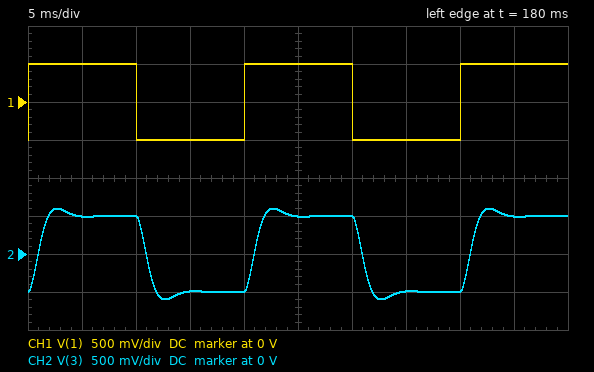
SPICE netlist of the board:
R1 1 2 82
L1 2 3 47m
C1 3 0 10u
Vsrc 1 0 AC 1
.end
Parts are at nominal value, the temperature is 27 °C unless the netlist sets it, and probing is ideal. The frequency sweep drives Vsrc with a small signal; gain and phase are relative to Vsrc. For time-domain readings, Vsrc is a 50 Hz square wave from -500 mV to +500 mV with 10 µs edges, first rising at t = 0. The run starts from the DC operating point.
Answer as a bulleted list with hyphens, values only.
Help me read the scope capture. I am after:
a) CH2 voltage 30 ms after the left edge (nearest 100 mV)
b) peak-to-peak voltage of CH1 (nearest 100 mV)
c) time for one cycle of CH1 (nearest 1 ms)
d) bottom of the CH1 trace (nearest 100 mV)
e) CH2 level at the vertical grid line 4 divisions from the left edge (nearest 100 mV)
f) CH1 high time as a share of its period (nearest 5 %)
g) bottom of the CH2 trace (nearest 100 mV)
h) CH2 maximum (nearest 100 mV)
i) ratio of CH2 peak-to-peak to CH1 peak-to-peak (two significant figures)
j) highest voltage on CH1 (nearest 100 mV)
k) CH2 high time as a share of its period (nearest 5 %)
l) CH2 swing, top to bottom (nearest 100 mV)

- 500 mV
- 1.0 V
- 20 ms
- -500 mV
- -500 mV
- 50 %
- -600 mV
- 600 mV
- 1.2
- 500 mV
- 50 %
- 1.2 V
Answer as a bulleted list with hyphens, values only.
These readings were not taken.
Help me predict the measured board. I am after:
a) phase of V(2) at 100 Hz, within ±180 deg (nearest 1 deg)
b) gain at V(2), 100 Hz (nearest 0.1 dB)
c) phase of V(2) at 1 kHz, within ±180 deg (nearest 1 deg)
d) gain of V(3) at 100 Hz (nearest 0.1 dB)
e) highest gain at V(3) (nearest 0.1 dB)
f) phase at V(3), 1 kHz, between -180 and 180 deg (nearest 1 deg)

- -32 deg
- -1.5 dB
- 16 deg
- 0.3 dB
- 0.4 dB
- -164 deg
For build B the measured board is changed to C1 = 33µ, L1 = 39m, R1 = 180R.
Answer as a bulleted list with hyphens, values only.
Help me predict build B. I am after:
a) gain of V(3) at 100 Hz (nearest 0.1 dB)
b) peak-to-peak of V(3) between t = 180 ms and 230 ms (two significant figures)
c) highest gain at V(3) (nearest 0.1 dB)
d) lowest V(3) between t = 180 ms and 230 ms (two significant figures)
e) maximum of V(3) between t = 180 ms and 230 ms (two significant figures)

- -11.5 dB
- 690 mV
- 0 dB
- -350 mV
- 350 mV
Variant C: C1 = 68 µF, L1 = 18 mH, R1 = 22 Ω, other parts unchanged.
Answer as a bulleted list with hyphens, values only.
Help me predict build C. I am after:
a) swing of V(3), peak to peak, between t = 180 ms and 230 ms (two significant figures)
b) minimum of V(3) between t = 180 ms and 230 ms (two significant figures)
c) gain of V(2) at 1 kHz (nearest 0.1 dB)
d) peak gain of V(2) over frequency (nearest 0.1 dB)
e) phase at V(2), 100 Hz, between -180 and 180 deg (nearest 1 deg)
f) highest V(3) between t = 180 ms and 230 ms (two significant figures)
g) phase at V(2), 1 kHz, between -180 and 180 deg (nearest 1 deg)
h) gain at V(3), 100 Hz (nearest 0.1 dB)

- 1.1 V
- -560 mV
- -0.2 dB
- 0 dB
- -61 deg
- 560 mV
- 11 deg
- -0.6 dB
